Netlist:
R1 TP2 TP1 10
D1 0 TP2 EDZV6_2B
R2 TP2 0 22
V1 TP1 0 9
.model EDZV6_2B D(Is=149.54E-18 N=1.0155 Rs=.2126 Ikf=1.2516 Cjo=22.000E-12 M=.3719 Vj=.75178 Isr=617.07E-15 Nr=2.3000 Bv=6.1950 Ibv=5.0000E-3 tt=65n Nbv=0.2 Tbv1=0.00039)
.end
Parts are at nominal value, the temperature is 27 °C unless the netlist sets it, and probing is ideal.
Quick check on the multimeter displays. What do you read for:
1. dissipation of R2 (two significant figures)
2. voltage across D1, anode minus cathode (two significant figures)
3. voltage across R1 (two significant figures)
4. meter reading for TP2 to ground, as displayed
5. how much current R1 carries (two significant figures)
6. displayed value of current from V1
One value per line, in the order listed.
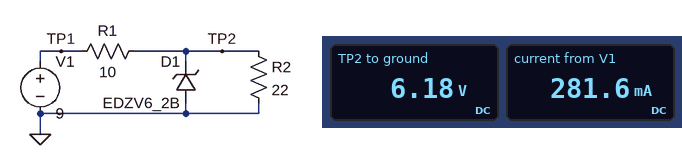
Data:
1.7 W
-6.2 V
2.8 V
6.18 V
280 mA
281.6 mA
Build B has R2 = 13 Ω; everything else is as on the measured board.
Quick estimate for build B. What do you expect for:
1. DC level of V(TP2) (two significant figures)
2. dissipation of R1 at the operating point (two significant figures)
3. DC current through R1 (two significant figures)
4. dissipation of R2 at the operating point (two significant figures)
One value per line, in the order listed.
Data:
5.1 V
1.5 W
390 mA
2.0 W
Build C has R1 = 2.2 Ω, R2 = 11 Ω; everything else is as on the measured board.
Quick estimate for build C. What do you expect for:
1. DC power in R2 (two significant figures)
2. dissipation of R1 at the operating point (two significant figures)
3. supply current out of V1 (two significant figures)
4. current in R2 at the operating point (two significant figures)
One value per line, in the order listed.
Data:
3.7 W
3.2 W
1.2 A
580 mA
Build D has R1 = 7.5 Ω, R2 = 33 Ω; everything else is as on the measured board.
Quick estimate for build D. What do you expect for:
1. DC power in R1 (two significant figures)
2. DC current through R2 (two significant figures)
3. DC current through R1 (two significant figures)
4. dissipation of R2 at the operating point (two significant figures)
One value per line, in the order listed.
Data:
1.0 W
190 mA
370 mA
1.2 W
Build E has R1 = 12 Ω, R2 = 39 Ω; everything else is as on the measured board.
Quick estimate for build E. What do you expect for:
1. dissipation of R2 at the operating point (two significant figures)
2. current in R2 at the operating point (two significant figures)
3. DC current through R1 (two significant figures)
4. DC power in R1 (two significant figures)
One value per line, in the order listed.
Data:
990 mW
160 mA
230 mA
640 mW
